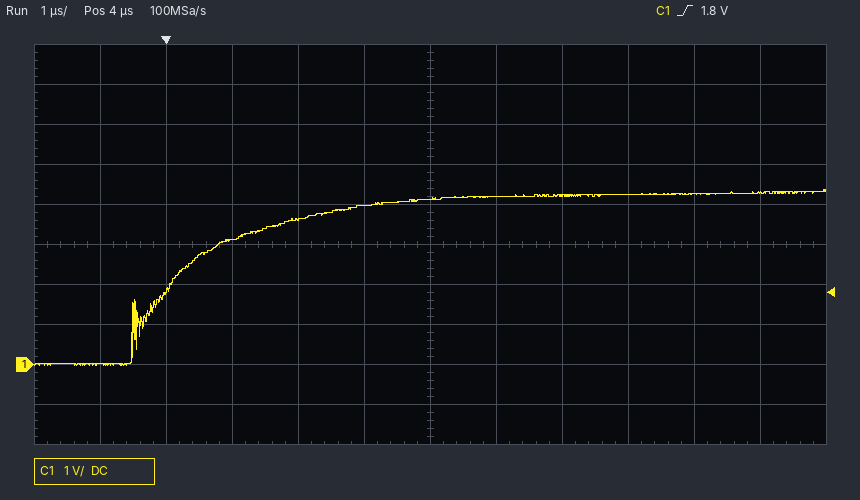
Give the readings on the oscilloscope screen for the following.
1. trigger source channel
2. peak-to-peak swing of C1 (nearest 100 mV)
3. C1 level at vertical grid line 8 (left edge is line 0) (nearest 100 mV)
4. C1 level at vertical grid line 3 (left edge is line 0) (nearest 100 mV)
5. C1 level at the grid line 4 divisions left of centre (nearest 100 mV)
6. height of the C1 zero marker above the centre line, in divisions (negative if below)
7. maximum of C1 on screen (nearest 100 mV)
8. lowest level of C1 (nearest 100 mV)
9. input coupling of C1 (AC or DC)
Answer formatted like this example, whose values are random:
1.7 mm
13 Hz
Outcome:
C1
4.4 V
4.2 V
3.1 V
1.8 V
-3.0 div
4.4 V
0.0 V
DC
